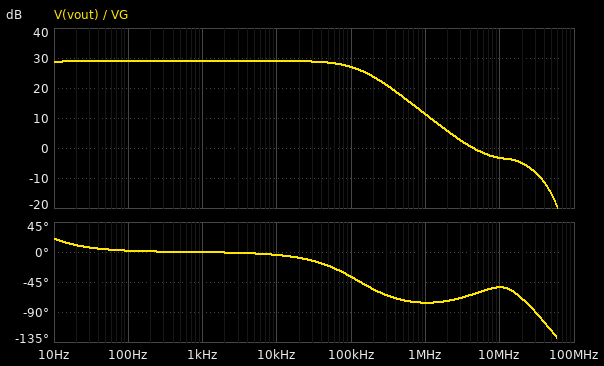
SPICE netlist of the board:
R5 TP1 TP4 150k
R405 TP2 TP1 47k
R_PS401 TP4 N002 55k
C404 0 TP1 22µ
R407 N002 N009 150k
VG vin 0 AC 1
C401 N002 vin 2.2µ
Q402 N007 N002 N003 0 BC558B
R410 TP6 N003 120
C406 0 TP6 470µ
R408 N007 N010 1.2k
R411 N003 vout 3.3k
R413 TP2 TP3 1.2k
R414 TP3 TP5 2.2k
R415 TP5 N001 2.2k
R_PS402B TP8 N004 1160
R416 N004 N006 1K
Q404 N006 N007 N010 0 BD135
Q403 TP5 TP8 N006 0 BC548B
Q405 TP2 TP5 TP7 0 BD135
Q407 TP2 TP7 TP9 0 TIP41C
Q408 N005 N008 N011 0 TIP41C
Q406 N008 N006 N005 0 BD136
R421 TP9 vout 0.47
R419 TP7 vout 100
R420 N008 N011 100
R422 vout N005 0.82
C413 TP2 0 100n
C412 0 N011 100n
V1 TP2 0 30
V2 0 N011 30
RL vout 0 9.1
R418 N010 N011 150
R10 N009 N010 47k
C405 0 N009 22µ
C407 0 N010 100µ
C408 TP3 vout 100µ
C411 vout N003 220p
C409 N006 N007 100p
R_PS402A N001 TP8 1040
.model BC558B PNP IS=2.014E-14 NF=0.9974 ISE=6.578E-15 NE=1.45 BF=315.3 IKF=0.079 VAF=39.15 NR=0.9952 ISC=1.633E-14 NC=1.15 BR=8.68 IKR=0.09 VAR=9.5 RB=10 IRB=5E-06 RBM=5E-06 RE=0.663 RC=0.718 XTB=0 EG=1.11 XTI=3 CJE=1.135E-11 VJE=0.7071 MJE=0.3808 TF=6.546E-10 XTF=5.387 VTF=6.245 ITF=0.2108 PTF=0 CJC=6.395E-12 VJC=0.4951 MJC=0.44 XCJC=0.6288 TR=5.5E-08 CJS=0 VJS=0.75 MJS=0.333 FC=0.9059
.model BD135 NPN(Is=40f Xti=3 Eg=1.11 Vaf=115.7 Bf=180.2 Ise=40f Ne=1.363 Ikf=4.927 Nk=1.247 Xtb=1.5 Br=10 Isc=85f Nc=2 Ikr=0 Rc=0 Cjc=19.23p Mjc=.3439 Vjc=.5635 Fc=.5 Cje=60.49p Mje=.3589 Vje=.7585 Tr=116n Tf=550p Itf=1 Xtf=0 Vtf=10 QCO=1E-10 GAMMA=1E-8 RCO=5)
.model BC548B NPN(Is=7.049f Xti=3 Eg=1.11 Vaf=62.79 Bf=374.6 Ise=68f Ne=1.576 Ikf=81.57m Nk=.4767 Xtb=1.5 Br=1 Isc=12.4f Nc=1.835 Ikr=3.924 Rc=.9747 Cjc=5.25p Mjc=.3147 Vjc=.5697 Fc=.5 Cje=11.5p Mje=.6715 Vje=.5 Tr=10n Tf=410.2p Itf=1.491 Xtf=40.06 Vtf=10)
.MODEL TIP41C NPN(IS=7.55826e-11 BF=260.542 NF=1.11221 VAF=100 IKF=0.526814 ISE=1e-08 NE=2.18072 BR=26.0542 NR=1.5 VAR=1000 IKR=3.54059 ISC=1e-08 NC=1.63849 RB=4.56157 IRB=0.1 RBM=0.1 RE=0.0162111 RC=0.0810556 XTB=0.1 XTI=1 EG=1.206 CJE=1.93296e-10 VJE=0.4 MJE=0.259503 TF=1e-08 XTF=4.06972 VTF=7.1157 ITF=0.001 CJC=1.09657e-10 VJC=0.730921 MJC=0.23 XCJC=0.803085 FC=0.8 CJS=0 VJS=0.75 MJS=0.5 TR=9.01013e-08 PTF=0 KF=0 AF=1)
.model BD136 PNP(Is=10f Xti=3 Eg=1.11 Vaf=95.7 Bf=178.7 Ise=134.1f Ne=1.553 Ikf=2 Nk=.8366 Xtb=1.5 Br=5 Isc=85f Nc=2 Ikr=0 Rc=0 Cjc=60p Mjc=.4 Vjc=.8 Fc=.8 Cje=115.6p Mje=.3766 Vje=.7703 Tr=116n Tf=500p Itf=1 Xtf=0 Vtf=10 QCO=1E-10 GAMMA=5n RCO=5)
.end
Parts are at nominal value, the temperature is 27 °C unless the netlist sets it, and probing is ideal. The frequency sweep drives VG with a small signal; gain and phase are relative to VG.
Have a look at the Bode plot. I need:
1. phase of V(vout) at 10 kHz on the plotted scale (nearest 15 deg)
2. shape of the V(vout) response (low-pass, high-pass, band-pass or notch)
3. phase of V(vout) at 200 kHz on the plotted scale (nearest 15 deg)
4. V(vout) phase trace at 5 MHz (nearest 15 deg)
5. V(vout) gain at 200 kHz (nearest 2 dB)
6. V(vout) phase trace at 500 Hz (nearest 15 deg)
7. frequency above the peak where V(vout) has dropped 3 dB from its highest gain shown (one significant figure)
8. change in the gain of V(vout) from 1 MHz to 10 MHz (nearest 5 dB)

0 deg
low-pass
-60 deg
-60 deg
24 dB
0 deg
100 kHz
-15 dB
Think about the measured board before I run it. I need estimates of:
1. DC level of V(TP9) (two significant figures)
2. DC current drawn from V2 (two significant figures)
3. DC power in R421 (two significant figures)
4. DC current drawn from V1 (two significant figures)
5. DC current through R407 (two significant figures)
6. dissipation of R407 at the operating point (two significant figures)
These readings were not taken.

-140 mV
35 mA
13 µW
19 mA
130 µA
2.6 mW
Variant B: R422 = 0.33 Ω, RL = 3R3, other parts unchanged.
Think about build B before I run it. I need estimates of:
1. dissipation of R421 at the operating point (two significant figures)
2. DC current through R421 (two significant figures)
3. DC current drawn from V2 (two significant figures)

14 µW
5.5 mA
64 mA
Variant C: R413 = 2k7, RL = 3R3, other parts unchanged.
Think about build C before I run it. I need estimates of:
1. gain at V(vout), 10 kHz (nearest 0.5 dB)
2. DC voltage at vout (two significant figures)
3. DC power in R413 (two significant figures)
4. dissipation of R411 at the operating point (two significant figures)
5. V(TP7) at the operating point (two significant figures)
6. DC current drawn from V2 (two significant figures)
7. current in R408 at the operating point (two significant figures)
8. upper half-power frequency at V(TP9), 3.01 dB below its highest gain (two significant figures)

29.0 dB
-430 mV
97 mW
1.1 mW
-56 mV
140 mA
550 µA
120 kHz
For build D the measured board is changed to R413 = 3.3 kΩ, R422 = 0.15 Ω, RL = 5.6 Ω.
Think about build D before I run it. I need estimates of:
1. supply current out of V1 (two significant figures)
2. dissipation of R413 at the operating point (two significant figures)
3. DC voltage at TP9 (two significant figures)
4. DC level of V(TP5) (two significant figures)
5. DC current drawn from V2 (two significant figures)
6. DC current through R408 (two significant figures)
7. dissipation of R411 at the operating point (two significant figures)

11 mA
94 mW
-510 mV
600 mV
100 mA
550 µA
1.1 mW
